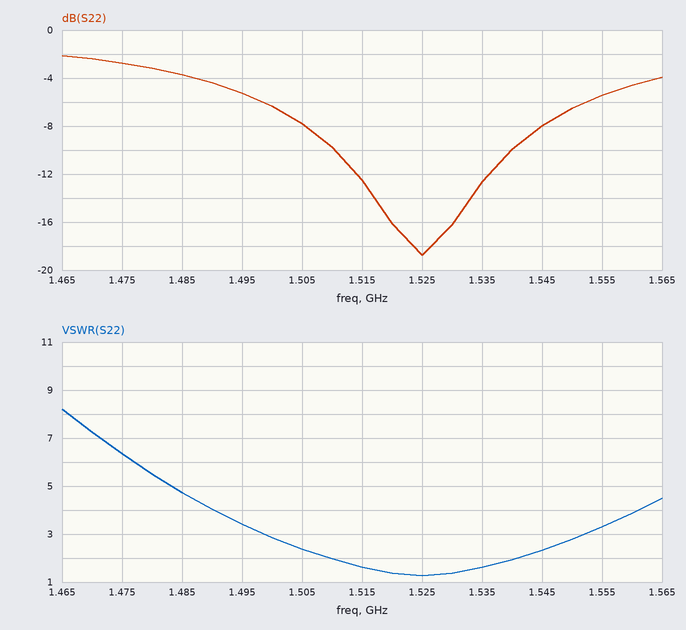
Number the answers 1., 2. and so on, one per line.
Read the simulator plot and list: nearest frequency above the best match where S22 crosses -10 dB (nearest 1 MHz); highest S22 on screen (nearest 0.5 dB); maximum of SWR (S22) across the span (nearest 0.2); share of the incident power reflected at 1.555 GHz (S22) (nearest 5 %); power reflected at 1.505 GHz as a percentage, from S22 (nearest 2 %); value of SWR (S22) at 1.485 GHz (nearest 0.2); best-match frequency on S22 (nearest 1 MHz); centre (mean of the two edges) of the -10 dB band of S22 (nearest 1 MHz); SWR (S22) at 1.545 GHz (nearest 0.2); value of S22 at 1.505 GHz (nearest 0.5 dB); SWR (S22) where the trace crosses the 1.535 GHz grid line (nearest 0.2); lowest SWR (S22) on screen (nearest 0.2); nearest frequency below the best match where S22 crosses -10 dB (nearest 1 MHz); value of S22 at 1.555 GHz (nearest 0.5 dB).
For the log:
1. 1.540 GHz
2. -2.0 dB
3. 8.2
4. 30 %
5. 16 %
6. 4.8
7. 1.525 GHz
8. 1.525 GHz
9. 2.4
10. -8.0 dB
11. 1.6
12. 1.2
13. 1.510 GHz
14. -5.5 dB
